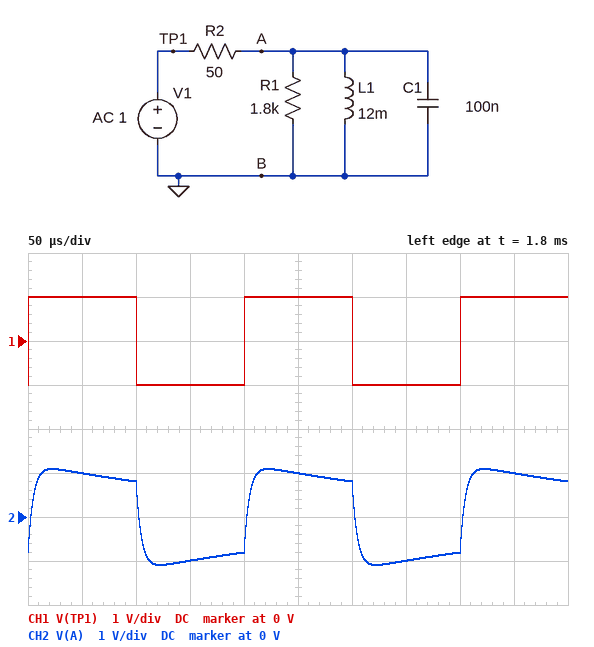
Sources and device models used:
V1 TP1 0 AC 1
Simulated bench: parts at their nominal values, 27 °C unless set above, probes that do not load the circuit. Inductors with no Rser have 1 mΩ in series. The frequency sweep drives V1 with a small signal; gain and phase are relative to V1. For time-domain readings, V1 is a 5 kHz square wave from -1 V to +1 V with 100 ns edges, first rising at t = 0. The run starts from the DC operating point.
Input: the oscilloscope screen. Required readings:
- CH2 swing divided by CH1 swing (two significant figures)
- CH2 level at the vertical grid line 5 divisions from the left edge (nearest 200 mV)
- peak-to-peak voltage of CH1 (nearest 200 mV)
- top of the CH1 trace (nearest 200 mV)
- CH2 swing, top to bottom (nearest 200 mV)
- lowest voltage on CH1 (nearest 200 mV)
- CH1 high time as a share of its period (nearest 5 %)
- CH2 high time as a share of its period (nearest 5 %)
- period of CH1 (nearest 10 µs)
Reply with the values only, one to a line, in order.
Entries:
1.1
1.0 V
2.0 V
1.0 V
2.2 V
-1.0 V
50 %
50 %
200 µs
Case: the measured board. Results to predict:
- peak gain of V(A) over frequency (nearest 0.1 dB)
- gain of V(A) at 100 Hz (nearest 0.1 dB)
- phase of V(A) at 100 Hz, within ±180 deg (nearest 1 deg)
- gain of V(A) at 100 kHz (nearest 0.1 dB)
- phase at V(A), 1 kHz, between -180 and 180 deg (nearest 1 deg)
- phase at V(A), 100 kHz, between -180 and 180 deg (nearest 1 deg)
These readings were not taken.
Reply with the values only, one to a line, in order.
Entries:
-0.2 dB
-16.5 dB
81 deg
-10.4 dB
32 deg
-72 deg
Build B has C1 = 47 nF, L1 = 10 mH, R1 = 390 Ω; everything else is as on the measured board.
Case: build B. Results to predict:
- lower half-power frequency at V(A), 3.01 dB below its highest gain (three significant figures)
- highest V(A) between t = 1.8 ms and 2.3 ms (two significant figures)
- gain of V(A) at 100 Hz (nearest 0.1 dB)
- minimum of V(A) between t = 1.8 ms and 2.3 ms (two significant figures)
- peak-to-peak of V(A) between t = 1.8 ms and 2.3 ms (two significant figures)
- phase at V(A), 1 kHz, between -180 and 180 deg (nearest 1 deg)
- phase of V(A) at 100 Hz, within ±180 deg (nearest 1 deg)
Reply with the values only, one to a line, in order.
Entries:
699 Hz
1.0 V
-18.1 dB
-1.0 V
2.1 V
35 deg
82 deg
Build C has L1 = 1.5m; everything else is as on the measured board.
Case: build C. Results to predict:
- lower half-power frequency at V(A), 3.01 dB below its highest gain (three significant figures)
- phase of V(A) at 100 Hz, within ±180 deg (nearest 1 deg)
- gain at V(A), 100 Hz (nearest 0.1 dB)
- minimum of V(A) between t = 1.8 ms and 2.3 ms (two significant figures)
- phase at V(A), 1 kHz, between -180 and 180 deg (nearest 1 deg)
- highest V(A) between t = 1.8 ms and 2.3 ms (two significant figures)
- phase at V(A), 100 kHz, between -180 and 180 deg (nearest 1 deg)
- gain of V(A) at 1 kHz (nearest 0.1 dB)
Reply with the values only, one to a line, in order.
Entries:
4.53 kHz
89 deg
-34.5 dB
-1.5 V
79 deg
1.5 V
-72 deg
-14.6 dB
